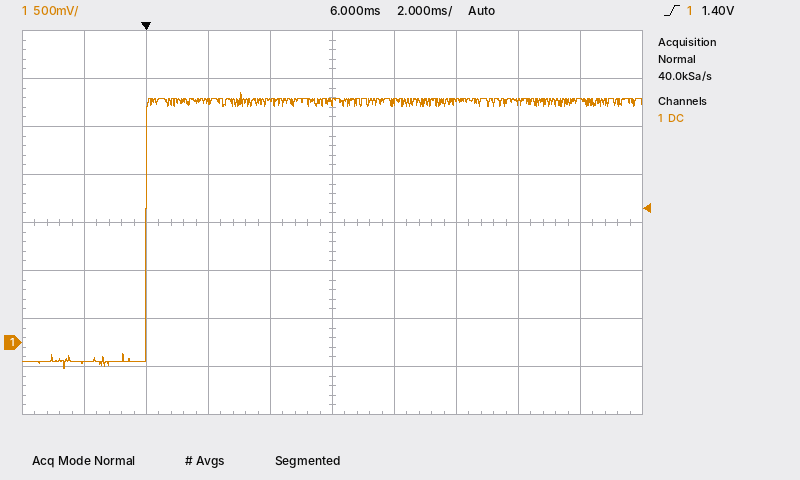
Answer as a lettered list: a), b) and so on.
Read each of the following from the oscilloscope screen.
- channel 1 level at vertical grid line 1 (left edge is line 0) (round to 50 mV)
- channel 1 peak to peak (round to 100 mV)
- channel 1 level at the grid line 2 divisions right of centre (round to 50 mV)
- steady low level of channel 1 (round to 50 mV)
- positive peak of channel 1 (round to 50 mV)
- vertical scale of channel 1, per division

a) -200 mV
b) 2.90 V
c) 2.50 V
d) -200 mV
e) 2.60 V
f) 500 mV
